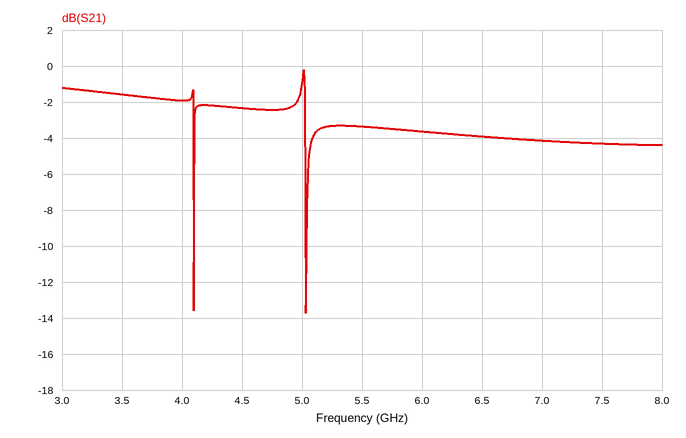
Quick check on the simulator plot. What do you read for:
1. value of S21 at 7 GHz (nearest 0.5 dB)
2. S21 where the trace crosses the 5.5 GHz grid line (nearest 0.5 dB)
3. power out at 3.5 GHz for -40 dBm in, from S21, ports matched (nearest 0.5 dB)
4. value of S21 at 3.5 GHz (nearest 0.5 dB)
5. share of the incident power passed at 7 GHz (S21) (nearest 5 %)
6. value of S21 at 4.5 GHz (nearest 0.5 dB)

-4.0 dB
-3.5 dB
-41.5 dBm
-1.5 dB
40 %
-2.5 dB
